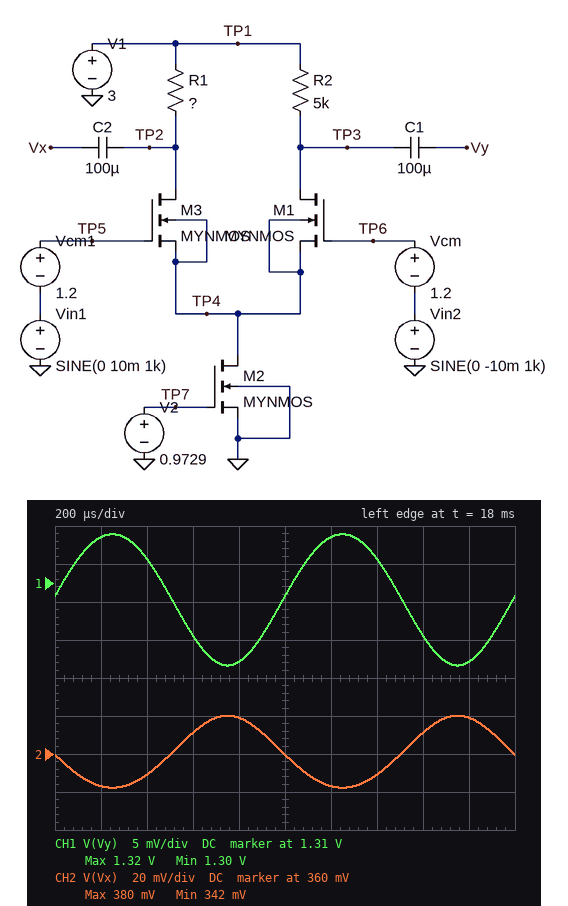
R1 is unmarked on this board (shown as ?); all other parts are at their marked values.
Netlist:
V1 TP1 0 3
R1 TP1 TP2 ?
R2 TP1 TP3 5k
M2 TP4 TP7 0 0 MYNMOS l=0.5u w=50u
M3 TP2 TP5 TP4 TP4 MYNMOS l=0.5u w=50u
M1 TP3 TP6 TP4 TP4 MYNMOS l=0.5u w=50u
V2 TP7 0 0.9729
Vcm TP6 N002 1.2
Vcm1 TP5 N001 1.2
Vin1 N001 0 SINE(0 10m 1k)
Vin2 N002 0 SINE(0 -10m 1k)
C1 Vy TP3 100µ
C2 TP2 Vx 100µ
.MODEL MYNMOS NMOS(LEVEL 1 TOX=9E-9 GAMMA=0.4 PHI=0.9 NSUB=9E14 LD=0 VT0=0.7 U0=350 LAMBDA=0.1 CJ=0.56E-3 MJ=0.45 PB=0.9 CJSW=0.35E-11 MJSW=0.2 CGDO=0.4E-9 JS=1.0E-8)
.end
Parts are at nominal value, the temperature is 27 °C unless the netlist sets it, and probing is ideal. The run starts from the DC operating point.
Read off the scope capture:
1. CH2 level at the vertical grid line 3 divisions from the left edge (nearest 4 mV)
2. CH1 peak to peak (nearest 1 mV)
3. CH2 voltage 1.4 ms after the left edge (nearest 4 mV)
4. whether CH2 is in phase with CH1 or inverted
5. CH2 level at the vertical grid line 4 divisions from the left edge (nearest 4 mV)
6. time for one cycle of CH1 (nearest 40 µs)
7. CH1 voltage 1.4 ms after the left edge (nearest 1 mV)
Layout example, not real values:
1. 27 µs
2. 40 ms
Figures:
1. 372 mV
2. 17 mV
3. 348 mV
4. inverted
5. 380 mV
6. 1.00 ms
7. 1.313 V
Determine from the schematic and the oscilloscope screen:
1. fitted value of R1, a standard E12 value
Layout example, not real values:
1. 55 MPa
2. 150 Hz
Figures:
1. 15 kΩ
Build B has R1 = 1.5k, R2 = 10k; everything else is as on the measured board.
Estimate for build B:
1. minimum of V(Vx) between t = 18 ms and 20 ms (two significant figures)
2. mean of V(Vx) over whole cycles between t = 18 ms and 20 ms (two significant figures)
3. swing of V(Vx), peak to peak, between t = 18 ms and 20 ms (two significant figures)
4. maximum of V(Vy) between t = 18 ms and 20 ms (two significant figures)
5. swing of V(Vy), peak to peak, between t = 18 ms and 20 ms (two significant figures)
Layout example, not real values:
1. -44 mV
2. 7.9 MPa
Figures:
1. 2.5 V
2. 2.6 V
3. 64 mV
4. 890 mV
5. 420 mV
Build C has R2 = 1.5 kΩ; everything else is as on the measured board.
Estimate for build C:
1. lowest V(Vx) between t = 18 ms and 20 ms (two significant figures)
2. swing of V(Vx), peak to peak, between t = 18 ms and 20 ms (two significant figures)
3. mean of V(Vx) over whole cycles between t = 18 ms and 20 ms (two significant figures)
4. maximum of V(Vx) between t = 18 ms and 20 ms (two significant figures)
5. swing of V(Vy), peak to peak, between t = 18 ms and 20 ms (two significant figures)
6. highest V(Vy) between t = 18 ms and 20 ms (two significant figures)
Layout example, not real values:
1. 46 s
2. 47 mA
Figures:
1. 360 mV
2. 42 mV
3. 380 mV
4. 400 mV
5. 5.6 mV
6. 2.5 V
